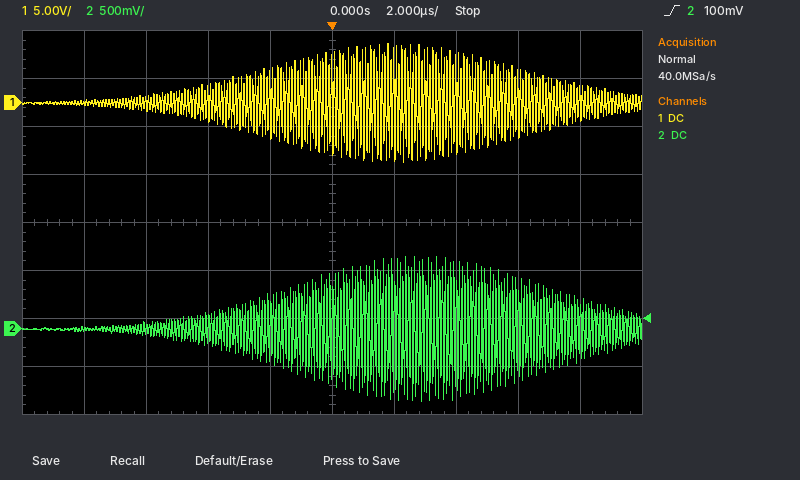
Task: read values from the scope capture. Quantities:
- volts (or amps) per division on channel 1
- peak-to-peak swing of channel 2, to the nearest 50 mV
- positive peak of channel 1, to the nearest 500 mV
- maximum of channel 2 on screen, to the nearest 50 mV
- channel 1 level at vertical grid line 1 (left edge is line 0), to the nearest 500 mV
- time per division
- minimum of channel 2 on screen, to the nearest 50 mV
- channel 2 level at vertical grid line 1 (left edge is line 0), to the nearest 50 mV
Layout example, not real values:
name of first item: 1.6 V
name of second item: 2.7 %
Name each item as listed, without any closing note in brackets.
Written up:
volts (or amps) per division on channel 1: 5 V
peak-to-peak swing of channel 2, to the nearest 50 mV: 1.50 V
positive peak of channel 1, to the nearest 500 mV: 6.0 V
maximum of channel 2 on screen, to the nearest 50 mV: 750 mV
channel 1 level at vertical grid line 1 (left edge is line 0), to the nearest 500 mV: 0.0 V
time per division: 2 µs
minimum of channel 2 on screen, to the nearest 50 mV: -750 mV
channel 2 level at vertical grid line 1 (left edge is line 0), to the nearest 50 mV: 0 mV
